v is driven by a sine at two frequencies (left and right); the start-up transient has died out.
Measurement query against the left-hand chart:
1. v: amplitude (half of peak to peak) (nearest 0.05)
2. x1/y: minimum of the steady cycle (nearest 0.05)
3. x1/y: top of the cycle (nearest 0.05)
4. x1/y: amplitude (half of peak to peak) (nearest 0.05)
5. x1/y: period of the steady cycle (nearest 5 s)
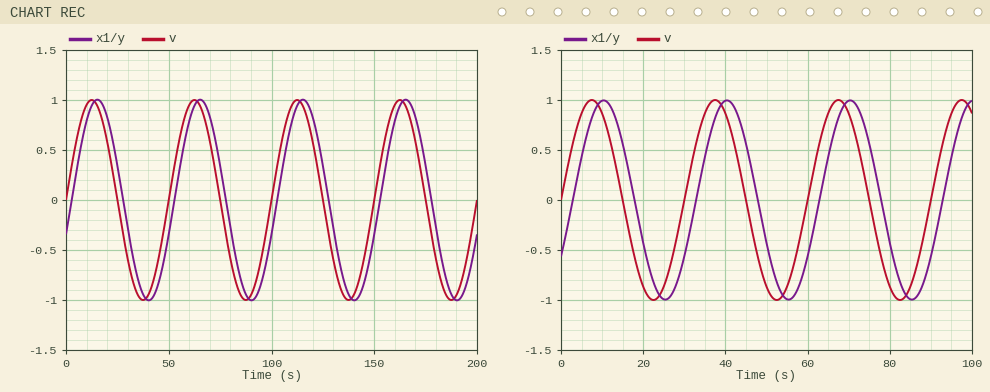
1.00
-1.00
1.00
1.00
50 s
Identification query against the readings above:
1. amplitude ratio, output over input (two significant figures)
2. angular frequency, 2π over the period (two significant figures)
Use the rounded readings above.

1.0
0.13 rad/s
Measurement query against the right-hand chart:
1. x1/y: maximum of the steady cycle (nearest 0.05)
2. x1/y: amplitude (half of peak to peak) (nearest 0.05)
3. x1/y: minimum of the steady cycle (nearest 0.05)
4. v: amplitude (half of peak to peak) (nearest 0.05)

1.00
1.00
-1.00
1.00
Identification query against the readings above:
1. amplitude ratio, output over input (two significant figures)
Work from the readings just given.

1.0
